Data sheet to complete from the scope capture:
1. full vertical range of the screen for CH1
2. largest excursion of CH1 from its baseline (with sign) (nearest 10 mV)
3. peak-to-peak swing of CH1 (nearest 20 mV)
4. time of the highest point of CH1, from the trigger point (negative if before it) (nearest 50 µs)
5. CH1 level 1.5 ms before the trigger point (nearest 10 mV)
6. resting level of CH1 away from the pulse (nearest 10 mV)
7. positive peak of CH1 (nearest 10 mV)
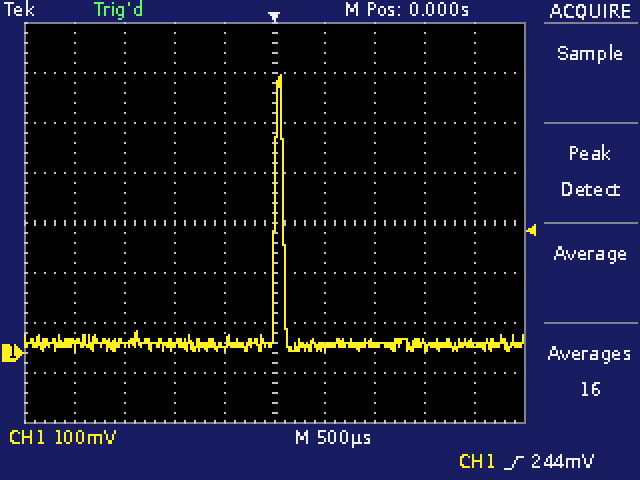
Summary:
800 mV
+540 mV
560 mV
+50 µs
20 mV
20 mV
560 mV
